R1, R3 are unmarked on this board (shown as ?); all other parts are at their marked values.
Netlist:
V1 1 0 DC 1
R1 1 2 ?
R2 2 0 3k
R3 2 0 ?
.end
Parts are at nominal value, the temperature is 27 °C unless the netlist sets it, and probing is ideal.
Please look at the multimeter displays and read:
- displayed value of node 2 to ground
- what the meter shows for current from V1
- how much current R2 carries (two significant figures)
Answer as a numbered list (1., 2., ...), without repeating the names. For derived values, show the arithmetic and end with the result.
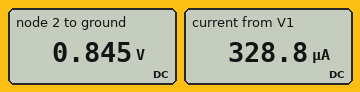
1. 0.845 V
2. 328.8 µA
3. (845 mV) / 3 kΩ = 280 µA
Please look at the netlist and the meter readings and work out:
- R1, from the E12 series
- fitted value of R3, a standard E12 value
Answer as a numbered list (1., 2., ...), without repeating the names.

1. 470 Ω
2. 18 kΩ
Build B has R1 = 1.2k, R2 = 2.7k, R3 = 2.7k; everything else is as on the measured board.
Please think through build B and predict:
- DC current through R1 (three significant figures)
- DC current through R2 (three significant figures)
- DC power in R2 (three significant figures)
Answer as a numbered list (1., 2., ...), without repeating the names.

1. 392 µA
2. 196 µA
3. 104 µW
